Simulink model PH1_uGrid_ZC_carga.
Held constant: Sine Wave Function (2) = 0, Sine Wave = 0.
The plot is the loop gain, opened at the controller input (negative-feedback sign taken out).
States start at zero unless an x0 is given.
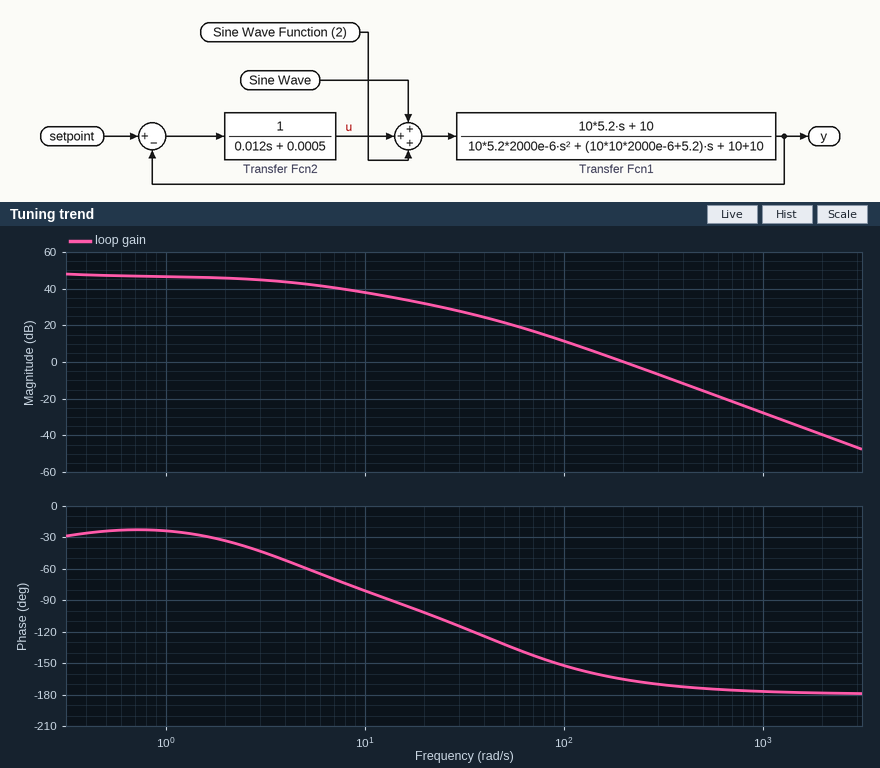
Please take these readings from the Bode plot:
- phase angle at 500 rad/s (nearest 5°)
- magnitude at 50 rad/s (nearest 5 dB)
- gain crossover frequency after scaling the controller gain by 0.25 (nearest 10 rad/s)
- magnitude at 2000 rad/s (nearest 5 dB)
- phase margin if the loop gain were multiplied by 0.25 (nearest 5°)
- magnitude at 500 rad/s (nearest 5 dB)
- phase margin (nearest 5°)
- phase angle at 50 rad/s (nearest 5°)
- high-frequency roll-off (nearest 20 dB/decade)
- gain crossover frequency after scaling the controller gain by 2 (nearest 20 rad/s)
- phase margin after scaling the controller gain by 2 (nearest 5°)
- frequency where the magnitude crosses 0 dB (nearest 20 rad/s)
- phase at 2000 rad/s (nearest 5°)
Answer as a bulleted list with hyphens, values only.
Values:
- -175°
- 20 dB
- 100 rad/s
- -40 dB
- 30°
- -15 dB
- 15°
- -130°
- -40 dB/decade
- 280 rad/s
- 10°
- 200 rad/s
- -180°
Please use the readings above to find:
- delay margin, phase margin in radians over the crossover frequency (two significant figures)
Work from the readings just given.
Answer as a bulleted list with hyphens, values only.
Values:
- 0.0013 s
